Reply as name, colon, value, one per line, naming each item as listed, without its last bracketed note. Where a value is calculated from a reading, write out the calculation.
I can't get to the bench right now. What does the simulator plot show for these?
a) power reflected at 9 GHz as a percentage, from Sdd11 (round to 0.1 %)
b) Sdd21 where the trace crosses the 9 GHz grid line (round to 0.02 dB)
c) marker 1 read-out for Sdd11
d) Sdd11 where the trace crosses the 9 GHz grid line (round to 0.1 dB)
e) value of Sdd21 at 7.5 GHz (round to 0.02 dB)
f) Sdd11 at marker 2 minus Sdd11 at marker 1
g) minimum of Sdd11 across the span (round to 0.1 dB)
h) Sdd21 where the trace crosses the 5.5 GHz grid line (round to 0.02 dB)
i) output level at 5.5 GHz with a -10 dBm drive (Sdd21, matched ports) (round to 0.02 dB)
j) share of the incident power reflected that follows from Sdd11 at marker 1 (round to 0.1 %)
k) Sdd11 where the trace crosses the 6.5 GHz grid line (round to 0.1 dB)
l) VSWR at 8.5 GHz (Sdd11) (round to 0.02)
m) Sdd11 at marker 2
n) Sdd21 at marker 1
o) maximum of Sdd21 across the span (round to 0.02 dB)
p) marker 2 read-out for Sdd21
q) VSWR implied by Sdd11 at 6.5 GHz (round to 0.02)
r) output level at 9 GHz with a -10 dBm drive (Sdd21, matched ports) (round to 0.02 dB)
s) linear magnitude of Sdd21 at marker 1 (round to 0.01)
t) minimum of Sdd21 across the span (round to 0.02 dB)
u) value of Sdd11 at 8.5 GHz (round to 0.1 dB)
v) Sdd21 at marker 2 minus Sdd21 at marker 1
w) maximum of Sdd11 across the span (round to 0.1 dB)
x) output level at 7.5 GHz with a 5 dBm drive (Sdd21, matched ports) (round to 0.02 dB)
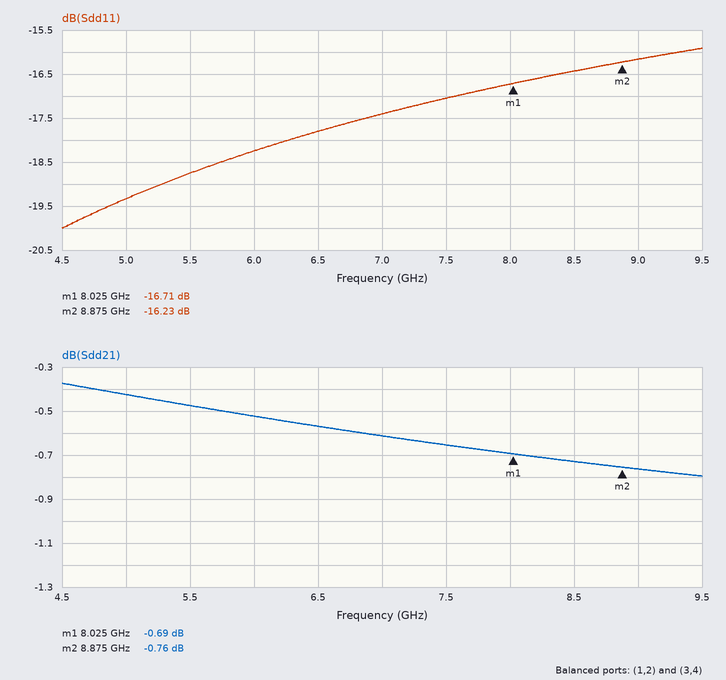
power reflected at 9 GHz as a percentage, from Sdd11: 10^(-16.2/10) ≈ 2.4 %
Sdd21 where the trace crosses the 9 GHz grid line: -0.76 dB
marker 1 read-out for Sdd11: -16.71 dB
Sdd11 where the trace crosses the 9 GHz grid line: -16.2 dB
value of Sdd21 at 7.5 GHz: -0.66 dB
Sdd11 at marker 2 minus Sdd11 at marker 1: -16.23 − (-16.71) = 0.48 dB
minimum of Sdd11 across the span: -20.0 dB
Sdd21 where the trace crosses the 5.5 GHz grid line: -0.48 dB
output level at 5.5 GHz with a -10 dBm drive (Sdd21, matched ports): -10 dBm + (-0.48 dB) = -10.48 dBm
share of the incident power reflected that follows from Sdd11 at marker 1: 10^(-16.71/10) ≈ 2.1 %
Sdd11 where the trace crosses the 6.5 GHz grid line: -17.8 dB
VSWR at 8.5 GHz (Sdd11): |Γ| = 10^(-16.4/20) = 0.1514; VSWR = (1 + 0.1514)/(1 − 0.1514) ≈ 1.36
Sdd11 at marker 2: -16.23 dB
Sdd21 at marker 1: -0.69 dB
maximum of Sdd21 across the span: -0.38 dB
marker 2 read-out for Sdd21: -0.76 dB
VSWR implied by Sdd11 at 6.5 GHz: |Γ| = 10^(-17.8/20) = 0.1288; VSWR = (1 + 0.1288)/(1 − 0.1288) ≈ 1.30
output level at 9 GHz with a -10 dBm drive (Sdd21, matched ports): -10 dBm + (-0.76 dB) = -10.76 dBm
linear magnitude of Sdd21 at marker 1: 10^(-0.69/20) ≈ 0.92
minimum of Sdd21 across the span: -0.80 dB
value of Sdd11 at 8.5 GHz: -16.4 dB
Sdd21 at marker 2 minus Sdd21 at marker 1: -0.76 − (-0.69) = -0.07 dB
maximum of Sdd11 across the span: -15.9 dB
output level at 7.5 GHz with a 5 dBm drive (Sdd21, matched ports): 5 dBm + (-0.66 dB) = 4.34 dBm
